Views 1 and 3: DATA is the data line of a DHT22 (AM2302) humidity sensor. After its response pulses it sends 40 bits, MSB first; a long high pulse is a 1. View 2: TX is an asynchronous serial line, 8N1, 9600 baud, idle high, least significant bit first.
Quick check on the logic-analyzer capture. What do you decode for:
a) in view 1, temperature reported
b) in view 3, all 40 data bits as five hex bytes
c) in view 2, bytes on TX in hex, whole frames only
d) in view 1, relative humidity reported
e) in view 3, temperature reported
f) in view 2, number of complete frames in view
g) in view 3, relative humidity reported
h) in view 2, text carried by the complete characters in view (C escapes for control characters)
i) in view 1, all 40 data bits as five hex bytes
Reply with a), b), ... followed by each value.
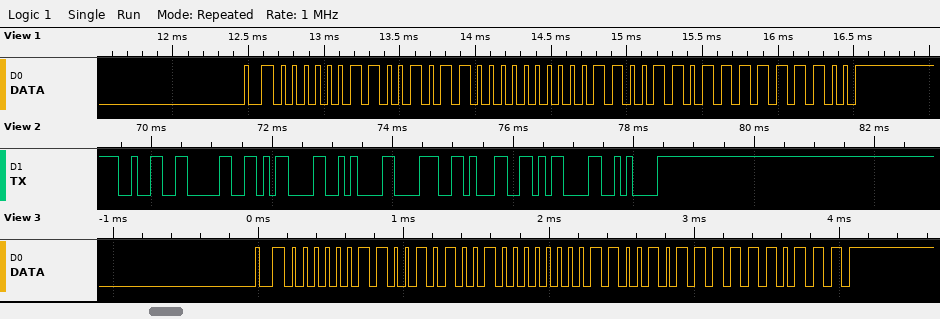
a) 20.5 °C
b) 03 29 00 CB F7
c) 32 30 0D 0A 38 31 0D 0A
d) 81.2 %
e) 20.3 °C
f) 8
g) 80.9 %
h) "20\r\n81\r\n"
i) 03 2C 00 CD FC
